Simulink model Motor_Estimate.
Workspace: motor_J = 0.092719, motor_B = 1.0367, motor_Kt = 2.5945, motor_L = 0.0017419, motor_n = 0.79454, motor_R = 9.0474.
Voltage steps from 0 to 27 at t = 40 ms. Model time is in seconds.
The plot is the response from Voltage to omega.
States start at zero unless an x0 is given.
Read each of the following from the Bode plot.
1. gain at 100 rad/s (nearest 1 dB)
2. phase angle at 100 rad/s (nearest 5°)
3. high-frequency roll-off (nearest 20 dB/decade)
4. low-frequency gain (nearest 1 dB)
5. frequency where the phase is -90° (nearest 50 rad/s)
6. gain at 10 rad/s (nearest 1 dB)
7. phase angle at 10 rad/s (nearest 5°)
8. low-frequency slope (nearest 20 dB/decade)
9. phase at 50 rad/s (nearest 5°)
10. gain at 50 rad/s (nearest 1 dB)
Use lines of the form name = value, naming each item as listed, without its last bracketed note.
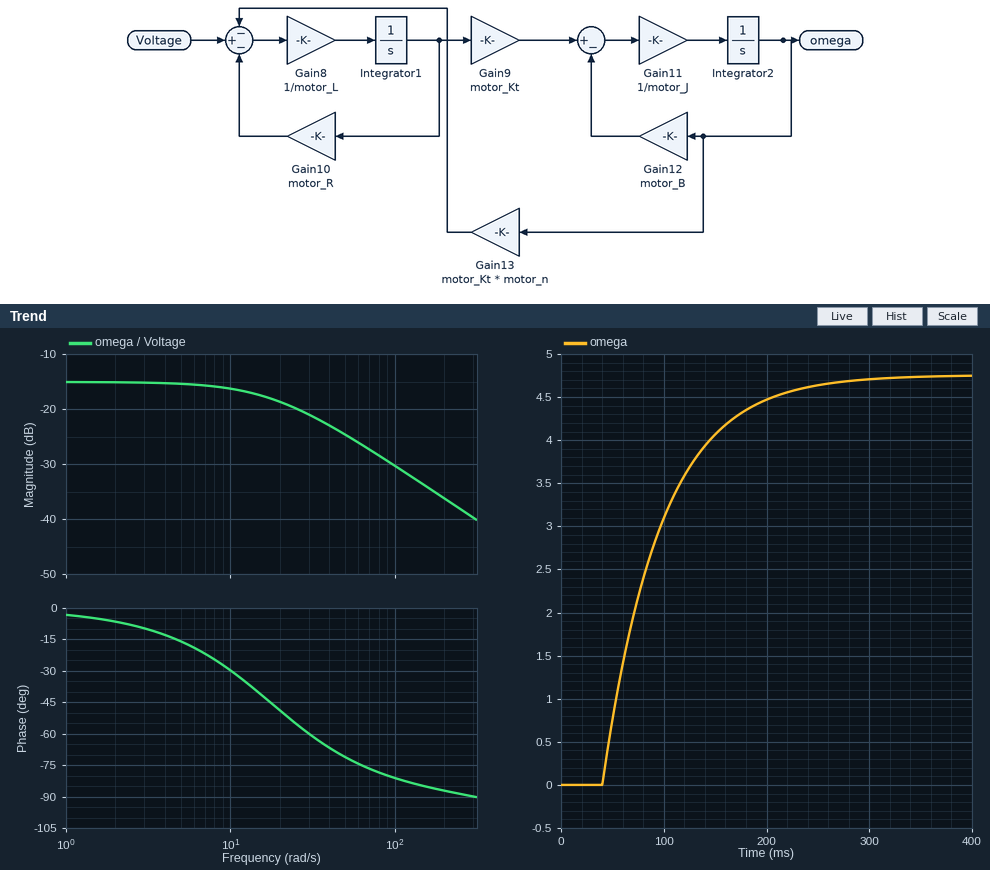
gain at 100 rad/s = -30 dB
phase angle at 100 rad/s = -80°
high-frequency roll-off = -20 dB/decade
low-frequency gain = -15 dB
frequency where the phase is -90° = 300 rad/s
gain at 10 rad/s = -16 dB
phase angle at 10 rad/s = -30°
low-frequency slope = 0 dB/decade
phase at 50 rad/s = -70°
gain at 50 rad/s = -25 dB
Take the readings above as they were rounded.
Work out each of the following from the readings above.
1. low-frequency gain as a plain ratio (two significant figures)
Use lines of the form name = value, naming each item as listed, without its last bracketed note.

low-frequency gain as a plain ratio = 0.18
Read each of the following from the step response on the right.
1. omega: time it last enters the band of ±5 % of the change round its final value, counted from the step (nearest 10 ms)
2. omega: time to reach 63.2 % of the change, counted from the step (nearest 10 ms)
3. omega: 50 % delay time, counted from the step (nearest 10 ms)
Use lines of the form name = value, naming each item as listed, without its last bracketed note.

omega: time it last enters the band of ±5 % of the change round its final value, counted from the step = 170 ms
omega: time to reach 63.2 % of the change, counted from the step = 60 ms
omega: 50 % delay time, counted from the step = 40 ms
